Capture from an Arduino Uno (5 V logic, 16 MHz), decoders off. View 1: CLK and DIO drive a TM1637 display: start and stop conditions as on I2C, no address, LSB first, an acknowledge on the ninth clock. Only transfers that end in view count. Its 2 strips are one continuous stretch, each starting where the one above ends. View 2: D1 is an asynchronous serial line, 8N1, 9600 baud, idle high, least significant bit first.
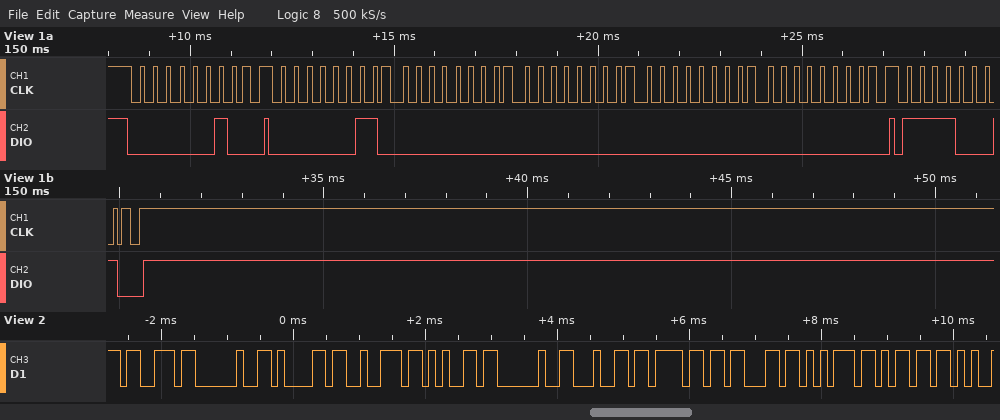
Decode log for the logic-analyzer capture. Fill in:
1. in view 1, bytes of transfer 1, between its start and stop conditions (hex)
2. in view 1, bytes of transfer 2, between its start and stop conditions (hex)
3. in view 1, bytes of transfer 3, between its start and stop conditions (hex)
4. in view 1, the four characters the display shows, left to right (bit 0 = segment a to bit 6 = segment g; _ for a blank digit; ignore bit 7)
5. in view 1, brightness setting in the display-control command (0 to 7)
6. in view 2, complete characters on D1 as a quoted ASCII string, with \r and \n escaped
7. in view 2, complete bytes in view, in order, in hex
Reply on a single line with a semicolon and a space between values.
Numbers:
40; C0 00 00 00 00; 8F; ____; 7; "s are docum"; 0x73 0x20 0x61 0x72 0x65 0x20 0x64 0x6F 0x63 0x75 0x6D
